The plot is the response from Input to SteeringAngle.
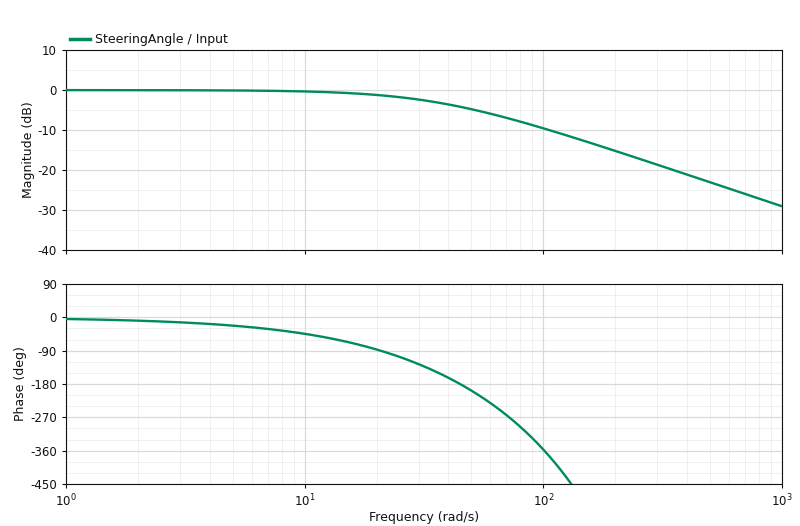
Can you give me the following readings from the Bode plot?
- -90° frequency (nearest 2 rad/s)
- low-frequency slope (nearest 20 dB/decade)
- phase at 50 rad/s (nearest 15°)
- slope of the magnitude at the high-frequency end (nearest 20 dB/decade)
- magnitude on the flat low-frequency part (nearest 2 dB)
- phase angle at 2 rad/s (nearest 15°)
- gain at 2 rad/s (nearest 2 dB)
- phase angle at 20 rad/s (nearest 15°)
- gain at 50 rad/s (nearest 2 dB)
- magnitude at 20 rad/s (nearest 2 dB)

20 rad/s
0 dB/decade
-195°
-20 dB/decade
0 dB
-15°
0 dB
-90°
-4 dB
-2 dB
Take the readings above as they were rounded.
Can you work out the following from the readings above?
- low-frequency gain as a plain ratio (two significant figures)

1.0
